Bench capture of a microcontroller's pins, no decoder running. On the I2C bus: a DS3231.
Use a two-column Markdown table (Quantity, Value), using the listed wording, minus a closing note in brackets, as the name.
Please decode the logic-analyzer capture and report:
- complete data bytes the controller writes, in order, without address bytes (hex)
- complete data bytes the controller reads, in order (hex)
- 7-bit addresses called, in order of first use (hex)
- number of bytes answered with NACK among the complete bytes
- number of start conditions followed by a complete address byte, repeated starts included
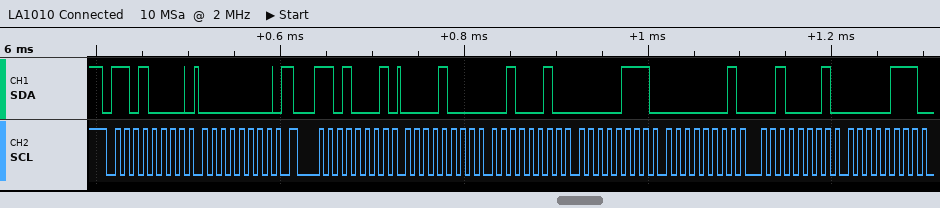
| Quantity | Value |
|---|---|
| complete data bytes the controller writes, in order, without address bytes | 00 |
| complete data bytes the controller reads, in order | 08 22 07 01 21 07 |
| 7-bit addresses called, in order of first use | 0x68 |
| number of bytes answered with NACK among the complete bytes | 0 |
| number of start conditions followed by a complete address byte, repeated starts included | 2 |
